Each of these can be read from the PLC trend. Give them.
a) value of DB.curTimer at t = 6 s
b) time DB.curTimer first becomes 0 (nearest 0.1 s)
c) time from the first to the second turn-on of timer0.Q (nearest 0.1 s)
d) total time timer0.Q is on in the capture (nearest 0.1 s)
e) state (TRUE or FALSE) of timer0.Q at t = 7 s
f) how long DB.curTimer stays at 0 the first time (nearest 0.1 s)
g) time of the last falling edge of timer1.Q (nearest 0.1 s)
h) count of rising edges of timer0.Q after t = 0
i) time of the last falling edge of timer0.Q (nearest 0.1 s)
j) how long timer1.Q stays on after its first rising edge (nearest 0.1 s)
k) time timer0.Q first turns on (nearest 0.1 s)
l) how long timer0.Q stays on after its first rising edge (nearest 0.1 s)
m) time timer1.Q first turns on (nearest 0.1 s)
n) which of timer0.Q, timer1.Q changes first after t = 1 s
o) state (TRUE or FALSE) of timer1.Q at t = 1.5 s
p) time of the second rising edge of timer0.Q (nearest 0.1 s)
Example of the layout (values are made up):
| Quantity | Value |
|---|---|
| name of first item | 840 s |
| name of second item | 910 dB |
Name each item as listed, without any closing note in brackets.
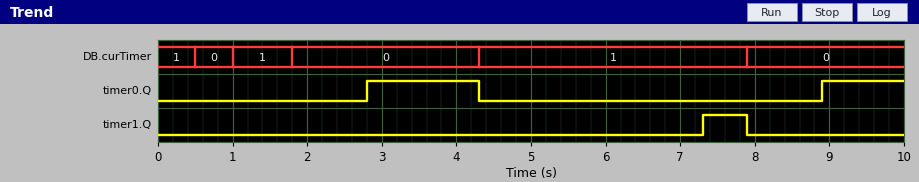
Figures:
| Quantity | Value |
|---|---|
| value of DB.curTimer at t = 6 s | 1 |
| time DB.curTimer first becomes 0 | 0.5 s |
| time from the first to the second turn-on of timer0.Q | 6.1 s |
| total time timer0.Q is on in the capture | 2.6 s |
| state (TRUE or FALSE) of timer0.Q at t = 7 s | FALSE |
| how long DB.curTimer stays at 0 the first time | 0.5 s |
| time of the last falling edge of timer1.Q | 7.9 s |
| count of rising edges of timer0.Q after t = 0 | 2 |
| time of the last falling edge of timer0.Q | 4.3 s |
| how long timer1.Q stays on after its first rising edge | 0.6 s |
| time timer0.Q first turns on | 2.8 s |
| how long timer0.Q stays on after its first rising edge | 1.5 s |
| time timer1.Q first turns on | 7.3 s |
| which of timer0.Q, timer1.Q changes first after t = 1 s | timer0.Q |
| state (TRUE or FALSE) of timer1.Q at t = 1.5 s | FALSE |
| time of the second rising edge of timer0.Q | 8.9 s |
